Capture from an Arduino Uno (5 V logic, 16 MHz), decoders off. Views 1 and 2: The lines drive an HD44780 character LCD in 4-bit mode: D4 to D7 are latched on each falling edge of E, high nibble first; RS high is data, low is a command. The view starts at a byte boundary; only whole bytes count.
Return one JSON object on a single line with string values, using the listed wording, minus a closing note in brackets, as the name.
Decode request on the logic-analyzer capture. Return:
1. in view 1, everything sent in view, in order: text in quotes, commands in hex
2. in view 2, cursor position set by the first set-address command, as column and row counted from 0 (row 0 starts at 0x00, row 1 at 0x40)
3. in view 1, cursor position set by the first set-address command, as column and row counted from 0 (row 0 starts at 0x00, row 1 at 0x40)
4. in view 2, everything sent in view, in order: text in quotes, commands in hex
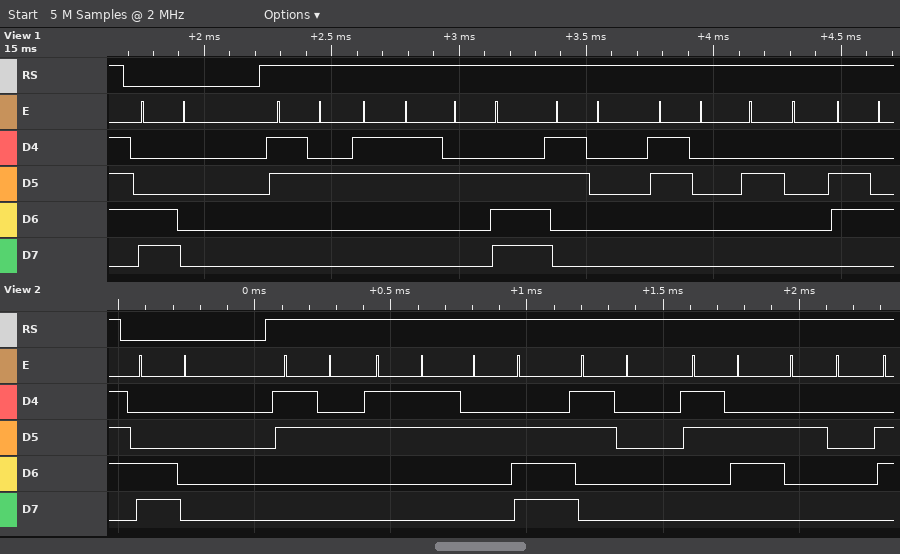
{"in view 1, everything sent in view, in order: text in quotes, commands in hex": "0xC0 \"23.00 d\"", "in view 2, cursor position set by the first set-address command, as column and row counted from 0": "column 0, row 1", "in view 1, cursor position set by the first set-address command, as column and row counted from 0": "column 0, row 1", "in view 2, everything sent in view, in order: text in quotes, commands in hex": "0xC0 \"23.06 \""}
